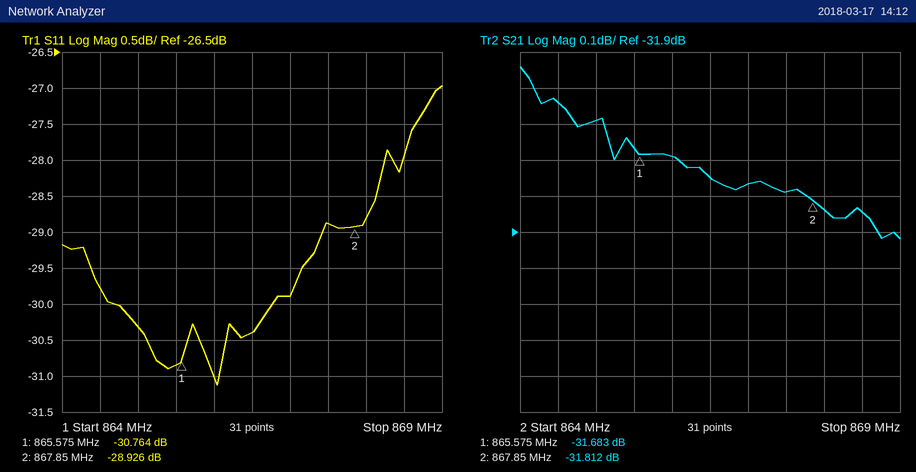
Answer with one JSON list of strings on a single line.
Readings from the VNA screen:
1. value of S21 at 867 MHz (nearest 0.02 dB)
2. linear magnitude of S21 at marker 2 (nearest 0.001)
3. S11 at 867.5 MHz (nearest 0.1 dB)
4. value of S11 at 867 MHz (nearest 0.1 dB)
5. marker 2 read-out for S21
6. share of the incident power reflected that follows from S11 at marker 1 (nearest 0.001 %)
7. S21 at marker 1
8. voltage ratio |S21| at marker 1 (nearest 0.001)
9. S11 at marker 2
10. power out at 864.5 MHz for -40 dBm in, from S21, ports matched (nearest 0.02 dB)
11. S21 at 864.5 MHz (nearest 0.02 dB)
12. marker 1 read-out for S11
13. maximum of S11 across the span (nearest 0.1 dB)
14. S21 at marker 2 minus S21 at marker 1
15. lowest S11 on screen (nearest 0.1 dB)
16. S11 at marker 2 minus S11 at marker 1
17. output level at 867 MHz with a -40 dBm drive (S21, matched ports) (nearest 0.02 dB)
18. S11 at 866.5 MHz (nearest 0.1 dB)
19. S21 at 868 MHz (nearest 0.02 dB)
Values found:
["-31.76 dB", "0.026", "-28.9 dB", "-29.9 dB", "-31.812 dB", "0.084 %", "-31.683 dB", "0.026", "-28.926 dB", "-71.54 dBm", "-31.54 dB", "-30.764 dB", "-27.0 dB", "-0.129 dB", "-31.1 dB", "1.838 dB", "-71.76 dBm", "-30.4 dB", "-31.84 dB"]
